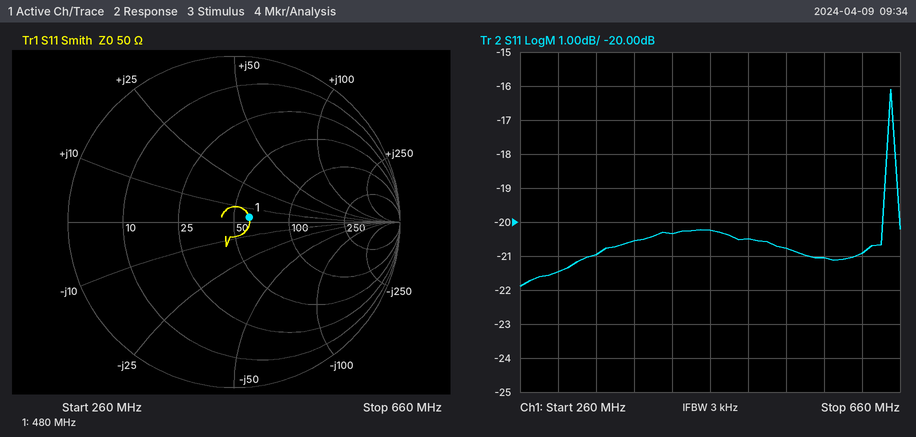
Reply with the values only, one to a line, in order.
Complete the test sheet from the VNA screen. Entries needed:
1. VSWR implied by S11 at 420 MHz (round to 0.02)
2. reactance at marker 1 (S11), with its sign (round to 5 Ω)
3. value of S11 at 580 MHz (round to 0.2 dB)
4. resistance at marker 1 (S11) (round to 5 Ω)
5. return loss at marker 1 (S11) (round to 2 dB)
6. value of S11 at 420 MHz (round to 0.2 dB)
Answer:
1.22
+5 Ω
-21.0 dB
60 Ω
20 dB
-20.4 dB
